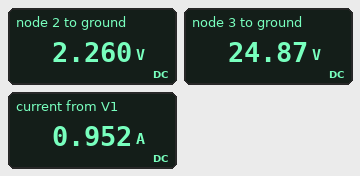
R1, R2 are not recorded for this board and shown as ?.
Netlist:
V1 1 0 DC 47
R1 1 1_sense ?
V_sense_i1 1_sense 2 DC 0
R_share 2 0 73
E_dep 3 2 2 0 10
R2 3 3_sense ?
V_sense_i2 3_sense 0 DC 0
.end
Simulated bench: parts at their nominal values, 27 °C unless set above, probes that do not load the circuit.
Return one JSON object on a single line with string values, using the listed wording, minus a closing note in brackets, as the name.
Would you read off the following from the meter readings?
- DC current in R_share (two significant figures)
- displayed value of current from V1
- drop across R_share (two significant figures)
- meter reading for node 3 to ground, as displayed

{"DC current in R_share": "31 mA", "displayed value of current from V1": "0.952 A", "drop across R_share": "2.3 V", "meter reading for node 3 to ground, as displayed": "24.87 V"}
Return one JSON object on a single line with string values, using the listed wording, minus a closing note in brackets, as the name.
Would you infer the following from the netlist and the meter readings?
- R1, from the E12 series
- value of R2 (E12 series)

{"R1, from the E12 series": "47 Ω", "value of R2": "27 Ω"}
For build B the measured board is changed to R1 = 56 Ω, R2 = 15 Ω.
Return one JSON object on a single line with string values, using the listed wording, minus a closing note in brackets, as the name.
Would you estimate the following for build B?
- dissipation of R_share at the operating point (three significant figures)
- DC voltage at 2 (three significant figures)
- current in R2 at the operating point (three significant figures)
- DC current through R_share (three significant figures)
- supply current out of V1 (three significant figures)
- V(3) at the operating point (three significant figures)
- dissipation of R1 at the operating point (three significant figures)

{"dissipation of R_share at the operating point": "16.5 mW", "DC voltage at 2": "1.10 V", "current in R2 at the operating point": "805 mA", "DC current through R_share": "15.0 mA", "supply current out of V1": "820 mA", "V(3) at the operating point": "12.1 V", "dissipation of R1 at the operating point": "37.6 W"}
